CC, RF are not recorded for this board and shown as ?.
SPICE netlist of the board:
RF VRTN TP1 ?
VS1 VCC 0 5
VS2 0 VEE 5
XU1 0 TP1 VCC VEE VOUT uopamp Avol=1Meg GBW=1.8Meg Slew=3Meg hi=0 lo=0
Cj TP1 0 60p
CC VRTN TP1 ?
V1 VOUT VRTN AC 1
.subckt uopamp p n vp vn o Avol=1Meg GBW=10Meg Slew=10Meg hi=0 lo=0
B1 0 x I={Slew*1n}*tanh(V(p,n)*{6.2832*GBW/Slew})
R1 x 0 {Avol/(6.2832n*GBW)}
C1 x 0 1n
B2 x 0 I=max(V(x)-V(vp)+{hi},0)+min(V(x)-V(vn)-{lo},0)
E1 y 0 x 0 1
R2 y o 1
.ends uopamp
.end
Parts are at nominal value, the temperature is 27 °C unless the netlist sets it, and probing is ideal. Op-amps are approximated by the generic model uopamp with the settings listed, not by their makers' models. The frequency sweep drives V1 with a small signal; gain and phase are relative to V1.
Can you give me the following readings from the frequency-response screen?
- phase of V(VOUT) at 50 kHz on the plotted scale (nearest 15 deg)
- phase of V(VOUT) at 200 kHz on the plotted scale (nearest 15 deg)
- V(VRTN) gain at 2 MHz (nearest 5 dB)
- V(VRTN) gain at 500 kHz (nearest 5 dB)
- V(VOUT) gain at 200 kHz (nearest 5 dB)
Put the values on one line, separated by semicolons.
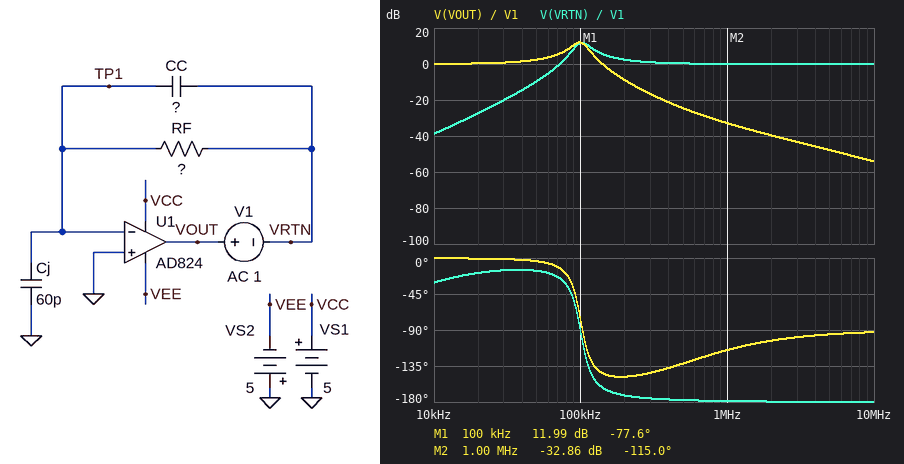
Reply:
0 deg; -150 deg; 0 dB; 0 dB; -10 dB
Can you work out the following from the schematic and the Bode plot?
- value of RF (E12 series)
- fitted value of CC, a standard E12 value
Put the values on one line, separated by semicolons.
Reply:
470 kΩ; 680 fF
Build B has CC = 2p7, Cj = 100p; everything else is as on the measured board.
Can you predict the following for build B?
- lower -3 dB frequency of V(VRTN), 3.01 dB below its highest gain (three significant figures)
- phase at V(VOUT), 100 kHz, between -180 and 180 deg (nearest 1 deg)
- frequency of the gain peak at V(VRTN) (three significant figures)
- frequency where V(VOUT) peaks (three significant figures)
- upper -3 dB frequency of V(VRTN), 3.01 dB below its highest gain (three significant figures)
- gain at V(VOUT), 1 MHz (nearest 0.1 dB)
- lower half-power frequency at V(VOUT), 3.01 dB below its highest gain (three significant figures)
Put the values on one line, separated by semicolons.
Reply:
65.0 kHz; -90 deg; 87.0 kHz; 70.6 kHz; 190 kHz; -26.4 dB; 40.0 kHz
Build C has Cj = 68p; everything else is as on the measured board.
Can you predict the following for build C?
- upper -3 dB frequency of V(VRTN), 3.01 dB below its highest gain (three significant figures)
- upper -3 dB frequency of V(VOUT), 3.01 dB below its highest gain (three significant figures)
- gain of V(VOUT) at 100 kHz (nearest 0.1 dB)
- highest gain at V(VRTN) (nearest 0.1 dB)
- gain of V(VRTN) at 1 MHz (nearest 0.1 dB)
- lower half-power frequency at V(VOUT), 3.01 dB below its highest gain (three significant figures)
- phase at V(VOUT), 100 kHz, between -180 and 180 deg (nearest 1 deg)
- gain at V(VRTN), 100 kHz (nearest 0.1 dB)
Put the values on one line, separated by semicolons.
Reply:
110 kHz; 104 kHz; 11.0 dB; 12.4 dB; 0.1 dB; 80.7 kHz; -105 deg; 11.9 dB
